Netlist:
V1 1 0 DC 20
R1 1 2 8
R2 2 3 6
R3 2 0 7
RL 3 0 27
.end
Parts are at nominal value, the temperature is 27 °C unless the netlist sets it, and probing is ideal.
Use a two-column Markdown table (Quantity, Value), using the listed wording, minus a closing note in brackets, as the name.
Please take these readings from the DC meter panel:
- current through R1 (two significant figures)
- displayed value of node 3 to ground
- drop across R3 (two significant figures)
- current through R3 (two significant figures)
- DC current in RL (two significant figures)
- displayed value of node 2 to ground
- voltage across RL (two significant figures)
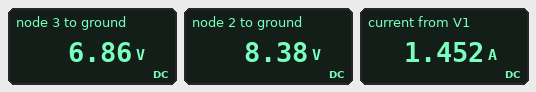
| Quantity | Value |
|---|---|
| current through R1 | 1.5 A |
| displayed value of node 3 to ground | 6.86 V |
| drop across R3 | 8.4 V |
| current through R3 | 1.2 A |
| DC current in RL | 250 mA |
| displayed value of node 2 to ground | 8.38 V |
| voltage across RL | 6.9 V |
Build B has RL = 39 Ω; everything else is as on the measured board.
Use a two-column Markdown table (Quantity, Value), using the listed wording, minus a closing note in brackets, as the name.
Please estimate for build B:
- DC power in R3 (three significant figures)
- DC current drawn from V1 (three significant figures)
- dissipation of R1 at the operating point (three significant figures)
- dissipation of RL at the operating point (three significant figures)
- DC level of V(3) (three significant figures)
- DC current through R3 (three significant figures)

| Quantity | Value |
|---|---|
| DC power in R3 | 10.6 W |
| DC current drawn from V1 | 1.42 A |
| dissipation of R1 at the operating point | 16.2 W |
| dissipation of RL at the operating point | 1.43 W |
| DC level of V(3) | 7.47 V |
| DC current through R3 | 1.23 A |
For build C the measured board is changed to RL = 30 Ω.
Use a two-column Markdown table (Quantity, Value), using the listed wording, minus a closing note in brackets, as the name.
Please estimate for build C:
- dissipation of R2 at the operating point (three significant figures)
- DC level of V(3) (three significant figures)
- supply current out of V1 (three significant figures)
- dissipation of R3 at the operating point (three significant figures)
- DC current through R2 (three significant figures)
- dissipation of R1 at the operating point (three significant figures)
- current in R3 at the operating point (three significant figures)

| Quantity | Value |
|---|---|
| dissipation of R2 at the operating point | 331 mW |
| DC level of V(3) | 7.05 V |
| supply current out of V1 | 1.44 A |
| dissipation of R3 at the operating point | 10.2 W |
| DC current through R2 | 235 mA |
| dissipation of R1 at the operating point | 16.7 W |
| current in R3 at the operating point | 1.21 A |
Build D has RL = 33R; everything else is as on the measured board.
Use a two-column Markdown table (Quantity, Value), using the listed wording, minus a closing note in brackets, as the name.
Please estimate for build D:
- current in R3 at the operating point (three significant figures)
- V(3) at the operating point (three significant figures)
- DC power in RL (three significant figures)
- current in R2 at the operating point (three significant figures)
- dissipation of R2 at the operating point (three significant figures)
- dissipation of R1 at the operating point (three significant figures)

| Quantity | Value |
|---|---|
| current in R3 at the operating point | 1.22 A |
| V(3) at the operating point | 7.21 V |
| DC power in RL | 1.57 W |
| current in R2 at the operating point | 218 mA |
| dissipation of R2 at the operating point | 286 mW |
| dissipation of R1 at the operating point | 16.5 W |
